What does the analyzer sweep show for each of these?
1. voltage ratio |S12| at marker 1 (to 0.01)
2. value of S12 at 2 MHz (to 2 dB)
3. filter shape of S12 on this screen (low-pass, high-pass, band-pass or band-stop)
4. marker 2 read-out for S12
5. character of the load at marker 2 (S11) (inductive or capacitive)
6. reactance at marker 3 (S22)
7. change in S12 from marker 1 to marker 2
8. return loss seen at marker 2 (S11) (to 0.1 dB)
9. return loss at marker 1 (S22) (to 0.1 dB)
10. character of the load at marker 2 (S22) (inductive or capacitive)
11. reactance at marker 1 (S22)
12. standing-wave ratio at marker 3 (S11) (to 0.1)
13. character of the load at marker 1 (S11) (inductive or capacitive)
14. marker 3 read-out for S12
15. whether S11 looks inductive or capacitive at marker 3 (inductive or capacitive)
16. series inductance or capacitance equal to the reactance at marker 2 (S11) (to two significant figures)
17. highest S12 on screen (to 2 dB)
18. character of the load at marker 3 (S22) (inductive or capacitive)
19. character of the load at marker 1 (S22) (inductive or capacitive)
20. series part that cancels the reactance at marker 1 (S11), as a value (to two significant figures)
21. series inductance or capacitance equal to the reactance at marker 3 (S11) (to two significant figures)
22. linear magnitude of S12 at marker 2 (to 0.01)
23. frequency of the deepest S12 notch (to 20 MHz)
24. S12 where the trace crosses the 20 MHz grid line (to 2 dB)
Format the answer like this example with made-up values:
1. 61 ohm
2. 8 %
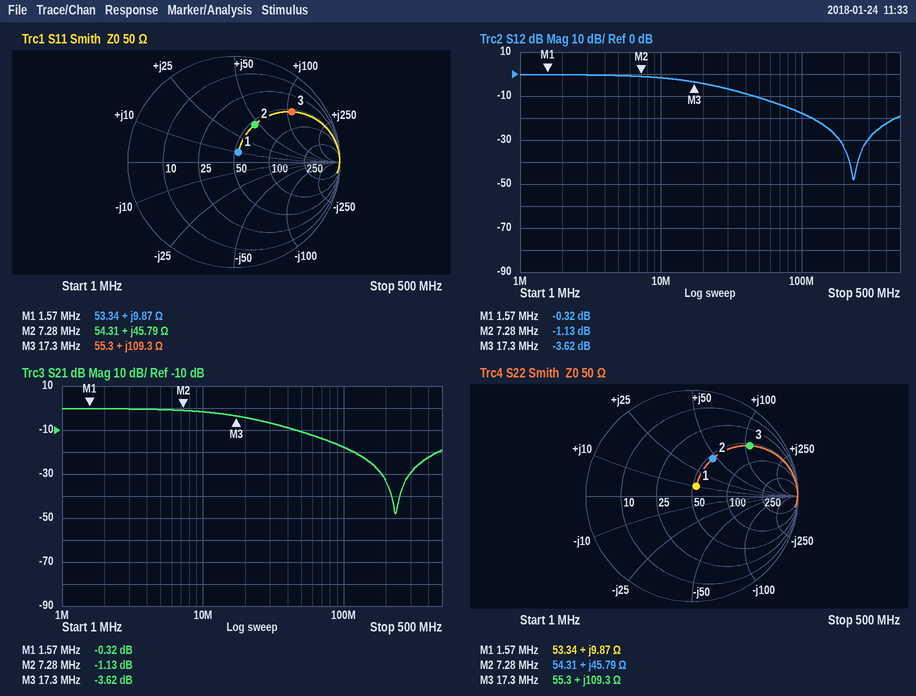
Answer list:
1. 0.96
2. 0 dB
3. low-pass
4. -1.13 dB
5. inductive
6. +109.3 Ω
7. -0.81 dB
8. 7.9 dB
9. 20.0 dB
10. inductive
11. +9.87 Ω
12. 6.2
13. inductive
14. -3.62 dB
15. inductive
16. 1.0 µH
17. 0 dB
18. inductive
19. inductive
20. 10 nF
21. 1.0 µH
22. 0.88
23. 240 MHz
24. -4 dB
